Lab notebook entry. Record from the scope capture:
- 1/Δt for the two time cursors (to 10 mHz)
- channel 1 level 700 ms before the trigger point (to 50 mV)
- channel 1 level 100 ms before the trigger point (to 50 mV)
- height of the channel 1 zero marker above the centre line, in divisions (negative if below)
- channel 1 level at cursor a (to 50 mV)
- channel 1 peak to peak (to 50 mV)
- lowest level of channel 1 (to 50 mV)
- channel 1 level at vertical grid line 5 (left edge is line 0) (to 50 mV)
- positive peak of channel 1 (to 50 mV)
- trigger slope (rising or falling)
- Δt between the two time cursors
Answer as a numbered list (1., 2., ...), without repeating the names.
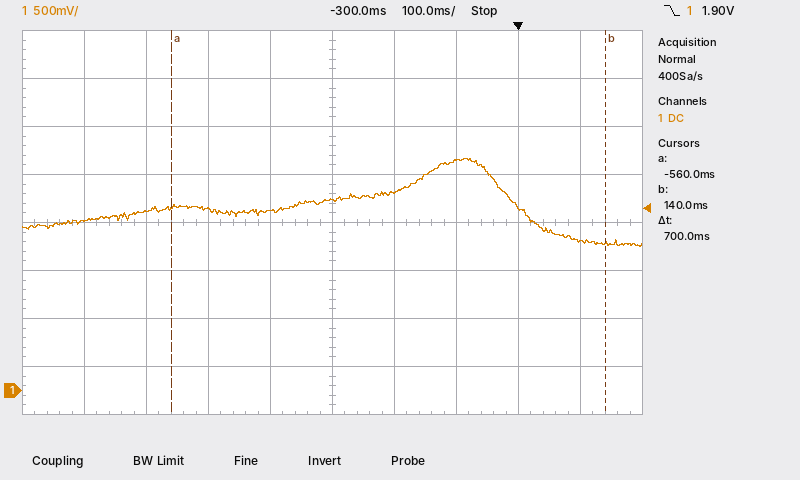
1. 1.43 Hz
2. 1.75 V
3. 2.40 V
4. -3.5 div
5. 1.90 V
6. 900 mV
7. 1.50 V
8. 2.00 V
9. 2.40 V
10. falling
11. 700 ms
